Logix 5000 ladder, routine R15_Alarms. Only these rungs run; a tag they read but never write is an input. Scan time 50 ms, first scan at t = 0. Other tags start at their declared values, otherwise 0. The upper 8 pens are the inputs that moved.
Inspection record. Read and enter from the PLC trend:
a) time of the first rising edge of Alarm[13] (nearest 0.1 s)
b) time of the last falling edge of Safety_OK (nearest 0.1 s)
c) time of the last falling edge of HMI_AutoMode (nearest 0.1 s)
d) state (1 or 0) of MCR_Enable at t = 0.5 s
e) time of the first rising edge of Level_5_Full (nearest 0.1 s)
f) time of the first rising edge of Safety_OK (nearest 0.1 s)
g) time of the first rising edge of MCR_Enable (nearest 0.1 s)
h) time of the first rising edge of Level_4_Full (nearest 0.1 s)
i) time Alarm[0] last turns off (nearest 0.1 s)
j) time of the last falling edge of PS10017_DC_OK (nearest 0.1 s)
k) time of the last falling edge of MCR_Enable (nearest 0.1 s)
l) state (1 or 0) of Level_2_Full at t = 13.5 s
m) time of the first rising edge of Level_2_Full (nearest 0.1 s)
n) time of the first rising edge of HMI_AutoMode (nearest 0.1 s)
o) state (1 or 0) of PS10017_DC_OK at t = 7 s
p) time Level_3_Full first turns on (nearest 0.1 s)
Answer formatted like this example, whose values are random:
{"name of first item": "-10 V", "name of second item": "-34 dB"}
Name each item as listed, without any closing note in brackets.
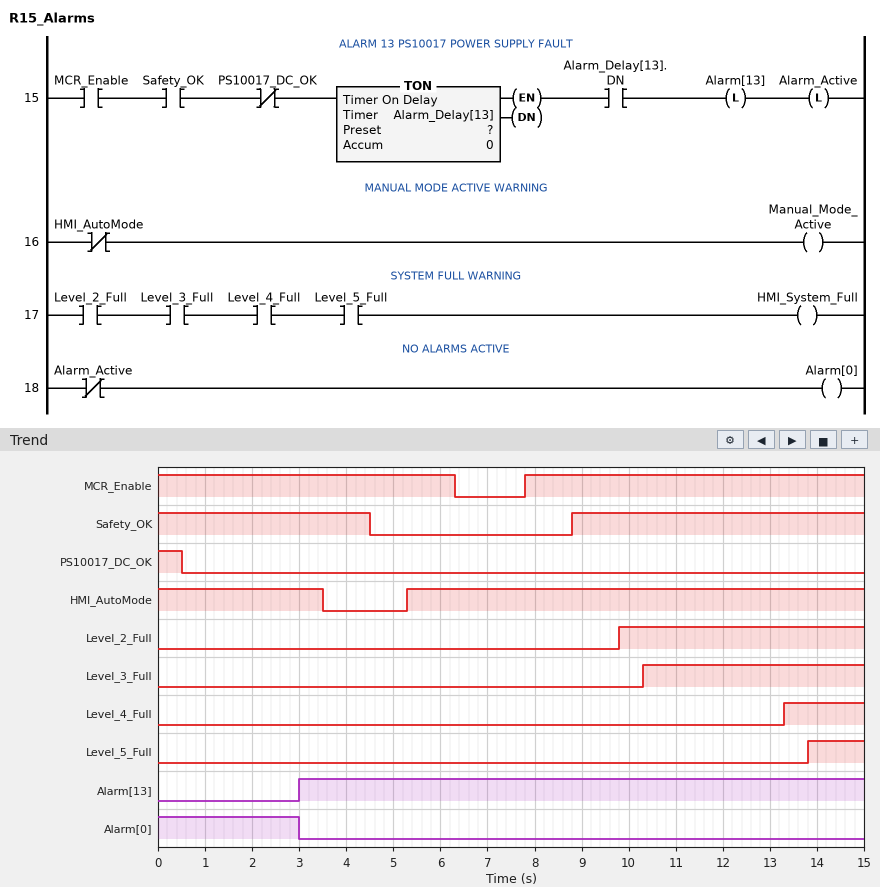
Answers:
{"time of the first rising edge of Alarm[13]": "3.0 s", "time of the last falling edge of Safety_OK": "4.5 s", "time of the last falling edge of HMI_AutoMode": "3.5 s", "state (1 or 0) of MCR_Enable at t = 0.5 s": "1", "time of the first rising edge of Level_5_Full": "13.8 s", "time of the first rising edge of Safety_OK": "8.8 s", "time of the first rising edge of MCR_Enable": "7.8 s", "time of the first rising edge of Level_4_Full": "13.3 s", "time Alarm[0] last turns off": "3.0 s", "time of the last falling edge of PS10017_DC_OK": "0.5 s", "time of the last falling edge of MCR_Enable": "6.3 s", "state (1 or 0) of Level_2_Full at t = 13.5 s": "1", "time of the first rising edge of Level_2_Full": "9.8 s", "time of the first rising edge of HMI_AutoMode": "5.3 s", "state (1 or 0) of PS10017_DC_OK at t = 7 s": "0", "time Level_3_Full first turns on": "10.3 s"}
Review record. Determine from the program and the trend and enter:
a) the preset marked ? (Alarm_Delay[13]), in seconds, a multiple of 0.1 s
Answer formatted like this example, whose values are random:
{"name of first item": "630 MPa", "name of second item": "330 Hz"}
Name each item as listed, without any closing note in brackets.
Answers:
{"the preset marked ? (Alarm_Delay[13]), in seconds, a multiple of 0.1 s": "2.5 s"}
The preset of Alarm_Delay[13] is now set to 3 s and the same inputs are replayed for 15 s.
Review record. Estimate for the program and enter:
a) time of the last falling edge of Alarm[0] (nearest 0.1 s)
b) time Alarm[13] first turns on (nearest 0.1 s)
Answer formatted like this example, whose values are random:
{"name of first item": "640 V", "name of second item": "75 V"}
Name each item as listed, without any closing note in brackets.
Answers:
{"time of the last falling edge of Alarm[0]": "3.5 s", "time Alarm[13] first turns on": "3.5 s"}
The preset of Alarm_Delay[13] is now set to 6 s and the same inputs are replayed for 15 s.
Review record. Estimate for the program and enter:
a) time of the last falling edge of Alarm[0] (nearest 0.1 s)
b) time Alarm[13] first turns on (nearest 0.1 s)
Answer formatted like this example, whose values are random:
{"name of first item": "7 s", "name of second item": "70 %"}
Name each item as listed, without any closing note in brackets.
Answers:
{"time of the last falling edge of Alarm[0]": "14.8 s", "time Alarm[13] first turns on": "14.8 s"}
